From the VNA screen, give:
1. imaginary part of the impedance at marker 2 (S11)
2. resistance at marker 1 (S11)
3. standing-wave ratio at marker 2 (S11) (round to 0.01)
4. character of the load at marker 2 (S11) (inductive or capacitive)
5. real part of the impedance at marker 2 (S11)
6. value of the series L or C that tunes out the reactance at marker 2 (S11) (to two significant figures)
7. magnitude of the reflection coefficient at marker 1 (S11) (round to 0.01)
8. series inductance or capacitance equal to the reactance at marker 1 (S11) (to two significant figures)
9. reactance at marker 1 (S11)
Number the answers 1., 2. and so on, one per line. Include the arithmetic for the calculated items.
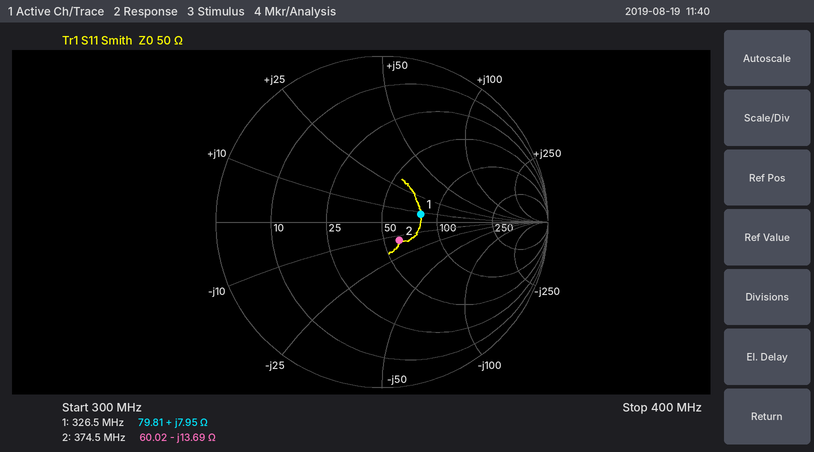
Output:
1. -13.69 Ω
2. 79.81 Ω
3. 1.36
4. capacitive
5. 60.02 Ω
6. L = 13.69 Ω/(2π × 374.5 MHz) ≈ 5.8 nH
7. 0.24
8. L = 7.95 Ω/(2π × 326.5 MHz) ≈ 3.9 nH
9. +7.95 Ω
